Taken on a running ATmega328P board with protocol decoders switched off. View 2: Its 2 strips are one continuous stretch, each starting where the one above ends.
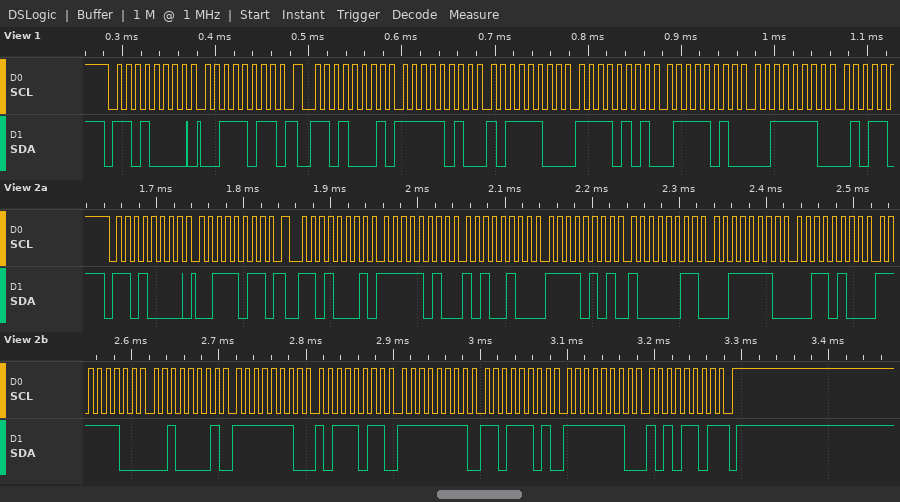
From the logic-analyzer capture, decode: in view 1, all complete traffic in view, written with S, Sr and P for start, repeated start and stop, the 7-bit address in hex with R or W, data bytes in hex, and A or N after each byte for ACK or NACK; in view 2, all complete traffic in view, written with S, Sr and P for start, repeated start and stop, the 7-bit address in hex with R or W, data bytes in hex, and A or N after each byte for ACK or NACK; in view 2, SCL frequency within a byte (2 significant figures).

S 68W A 3B A Sr 68R A FA A BC A F5 A 7A A 3E A
S 68W A 3B A Sr 68R A FA A A4 A F5 A 83 A 3E A 34 A FC A 21 A FE A BB A FF A DD A FE A AD N P
100 kHz
